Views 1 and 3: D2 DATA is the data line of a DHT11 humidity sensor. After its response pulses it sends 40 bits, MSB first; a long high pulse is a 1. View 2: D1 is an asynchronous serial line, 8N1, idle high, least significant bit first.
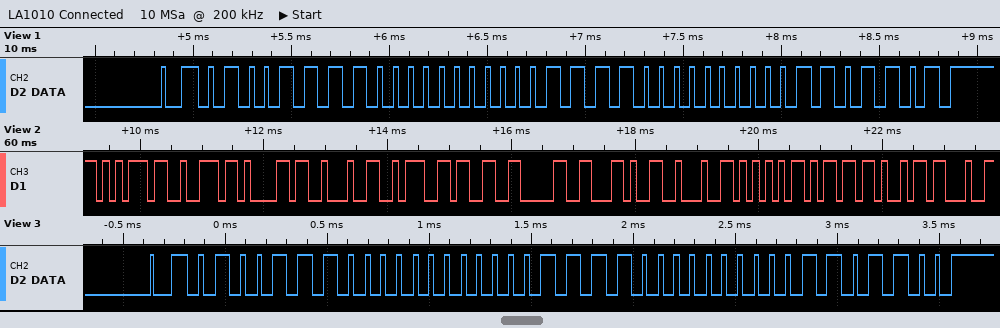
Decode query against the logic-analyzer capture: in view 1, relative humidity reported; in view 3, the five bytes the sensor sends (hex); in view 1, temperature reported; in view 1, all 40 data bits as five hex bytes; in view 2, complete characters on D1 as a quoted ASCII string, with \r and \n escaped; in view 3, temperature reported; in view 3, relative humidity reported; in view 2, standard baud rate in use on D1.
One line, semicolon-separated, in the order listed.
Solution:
79 %; 4E 00 1E 00 6C; 30.0 °C; 4F 00 1E 00 6D; "ura\":30,\"Umi"; 30.0 °C; 78 %; 9600 baud
